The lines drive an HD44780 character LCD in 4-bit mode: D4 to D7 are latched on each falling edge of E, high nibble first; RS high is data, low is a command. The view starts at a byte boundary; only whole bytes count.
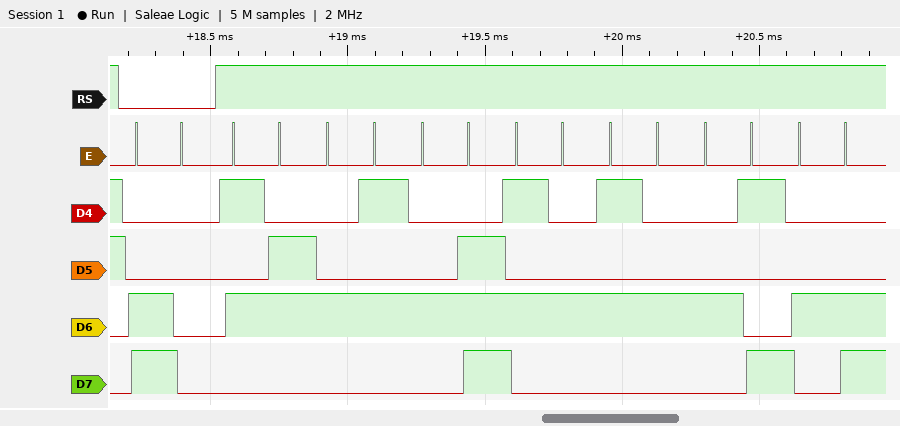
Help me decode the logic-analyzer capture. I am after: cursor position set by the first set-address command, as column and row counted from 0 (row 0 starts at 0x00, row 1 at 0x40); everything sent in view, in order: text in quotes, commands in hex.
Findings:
column 0, row 1
0xC0 "VENTTIL"
